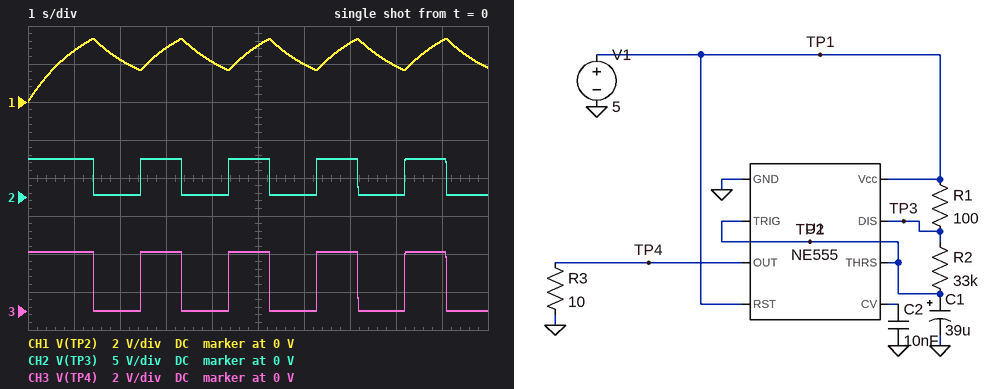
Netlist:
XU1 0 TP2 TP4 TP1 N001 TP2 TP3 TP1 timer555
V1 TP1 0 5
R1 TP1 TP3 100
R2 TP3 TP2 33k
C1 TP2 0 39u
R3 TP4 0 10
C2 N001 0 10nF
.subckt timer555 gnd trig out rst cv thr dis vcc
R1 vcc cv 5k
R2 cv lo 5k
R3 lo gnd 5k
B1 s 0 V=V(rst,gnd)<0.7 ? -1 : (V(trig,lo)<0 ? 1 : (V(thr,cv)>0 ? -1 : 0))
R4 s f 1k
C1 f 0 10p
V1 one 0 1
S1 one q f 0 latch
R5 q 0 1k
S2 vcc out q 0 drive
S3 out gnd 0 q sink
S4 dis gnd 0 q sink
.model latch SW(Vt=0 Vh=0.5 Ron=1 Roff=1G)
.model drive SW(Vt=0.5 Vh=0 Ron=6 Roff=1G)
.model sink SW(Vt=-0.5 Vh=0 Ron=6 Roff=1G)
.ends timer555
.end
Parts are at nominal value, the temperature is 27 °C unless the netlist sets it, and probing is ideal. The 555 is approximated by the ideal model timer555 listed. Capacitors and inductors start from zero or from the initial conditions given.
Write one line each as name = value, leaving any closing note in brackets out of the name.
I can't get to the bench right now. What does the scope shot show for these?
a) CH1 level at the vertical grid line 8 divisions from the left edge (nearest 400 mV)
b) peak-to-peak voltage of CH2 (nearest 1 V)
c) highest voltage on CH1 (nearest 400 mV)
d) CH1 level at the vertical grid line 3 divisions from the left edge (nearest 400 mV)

CH1 level at the vertical grid line 8 divisions from the left edge = 2.0 V
peak-to-peak voltage of CH2 = 5 V
highest voltage on CH1 = 3.2 V
CH1 level at the vertical grid line 3 divisions from the left edge = 2.8 V
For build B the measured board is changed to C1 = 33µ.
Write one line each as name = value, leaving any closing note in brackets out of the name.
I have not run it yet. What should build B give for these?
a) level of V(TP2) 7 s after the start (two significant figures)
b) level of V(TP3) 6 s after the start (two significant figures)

level of V(TP2) 7 s after the start = 1.9 V
level of V(TP3) 6 s after the start = 5.0 V
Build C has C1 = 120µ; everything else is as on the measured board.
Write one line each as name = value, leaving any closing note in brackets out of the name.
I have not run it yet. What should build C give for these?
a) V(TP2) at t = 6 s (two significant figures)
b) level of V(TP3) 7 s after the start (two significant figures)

V(TP2) at t = 6 s = 2.3 V
level of V(TP3) 7 s after the start = 280 mV
